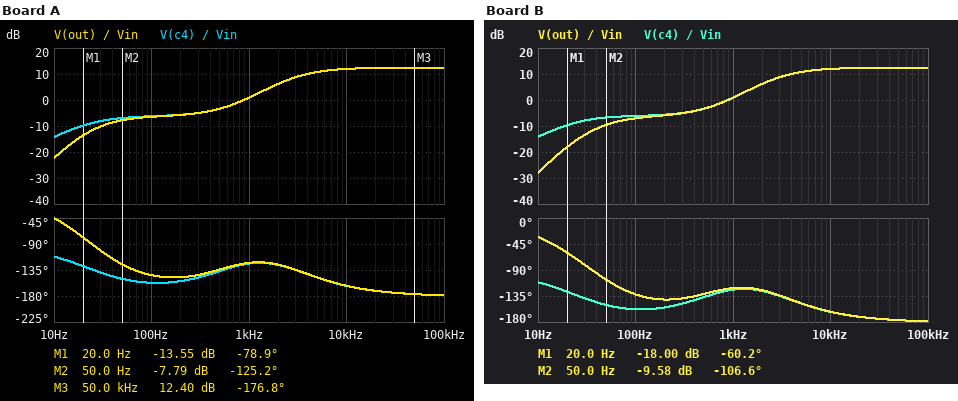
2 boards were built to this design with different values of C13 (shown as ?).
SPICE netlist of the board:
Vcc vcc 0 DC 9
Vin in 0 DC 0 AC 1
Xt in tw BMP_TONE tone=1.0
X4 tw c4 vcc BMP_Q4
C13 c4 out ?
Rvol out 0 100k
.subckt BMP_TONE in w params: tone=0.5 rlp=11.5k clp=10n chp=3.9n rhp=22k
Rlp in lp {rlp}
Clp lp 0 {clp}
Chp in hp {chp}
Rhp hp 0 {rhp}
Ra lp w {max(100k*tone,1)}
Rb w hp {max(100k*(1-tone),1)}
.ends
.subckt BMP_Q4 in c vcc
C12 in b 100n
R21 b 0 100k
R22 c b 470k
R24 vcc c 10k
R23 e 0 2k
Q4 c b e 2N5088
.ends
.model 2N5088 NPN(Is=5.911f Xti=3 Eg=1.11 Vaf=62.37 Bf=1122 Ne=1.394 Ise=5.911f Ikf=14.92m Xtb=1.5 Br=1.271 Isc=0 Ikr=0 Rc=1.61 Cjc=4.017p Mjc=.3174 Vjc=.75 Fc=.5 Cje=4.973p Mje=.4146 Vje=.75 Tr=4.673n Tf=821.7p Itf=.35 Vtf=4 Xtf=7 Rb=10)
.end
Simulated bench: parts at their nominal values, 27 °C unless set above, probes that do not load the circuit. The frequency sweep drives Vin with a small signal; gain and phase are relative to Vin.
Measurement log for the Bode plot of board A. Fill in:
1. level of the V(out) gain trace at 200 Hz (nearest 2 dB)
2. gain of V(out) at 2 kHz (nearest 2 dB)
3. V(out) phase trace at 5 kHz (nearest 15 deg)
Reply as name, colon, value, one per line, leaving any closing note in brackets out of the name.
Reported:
level of the V(out) gain trace at 200 Hz: -6 dB
gain of V(out) at 2 kHz: 6 dB
V(out) phase trace at 5 kHz: -150 deg
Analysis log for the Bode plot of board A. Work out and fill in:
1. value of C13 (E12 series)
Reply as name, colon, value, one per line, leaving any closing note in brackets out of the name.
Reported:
value of C13: 68 nF
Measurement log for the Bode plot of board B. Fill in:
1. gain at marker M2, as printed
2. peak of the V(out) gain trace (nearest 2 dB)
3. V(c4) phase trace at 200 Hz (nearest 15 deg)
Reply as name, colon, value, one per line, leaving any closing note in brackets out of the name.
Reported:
gain at marker M2, as printed: -9.58 dB
peak of the V(out) gain trace: 12 dB
V(c4) phase trace at 200 Hz: -150 deg
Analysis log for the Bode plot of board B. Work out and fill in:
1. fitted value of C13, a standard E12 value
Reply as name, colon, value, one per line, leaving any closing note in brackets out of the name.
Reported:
fitted value of C13, a standard E12 value: 33 nF
